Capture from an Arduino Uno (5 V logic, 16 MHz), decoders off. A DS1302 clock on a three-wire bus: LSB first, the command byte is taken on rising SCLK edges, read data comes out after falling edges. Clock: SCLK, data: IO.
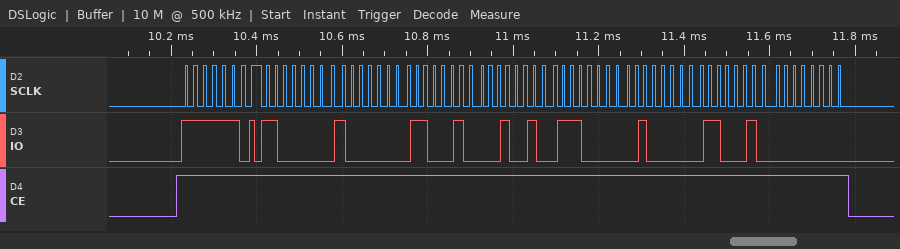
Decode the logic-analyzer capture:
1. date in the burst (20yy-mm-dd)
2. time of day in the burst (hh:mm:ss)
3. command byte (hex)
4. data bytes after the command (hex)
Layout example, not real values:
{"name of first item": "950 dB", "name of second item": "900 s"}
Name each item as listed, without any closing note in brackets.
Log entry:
{"date in the burst": "2023-07-24", "time of day in the burst": "23:01:03", "command byte": "0xBF", "data bytes after the command": "03 01 23 24 07 02 23 00"}
